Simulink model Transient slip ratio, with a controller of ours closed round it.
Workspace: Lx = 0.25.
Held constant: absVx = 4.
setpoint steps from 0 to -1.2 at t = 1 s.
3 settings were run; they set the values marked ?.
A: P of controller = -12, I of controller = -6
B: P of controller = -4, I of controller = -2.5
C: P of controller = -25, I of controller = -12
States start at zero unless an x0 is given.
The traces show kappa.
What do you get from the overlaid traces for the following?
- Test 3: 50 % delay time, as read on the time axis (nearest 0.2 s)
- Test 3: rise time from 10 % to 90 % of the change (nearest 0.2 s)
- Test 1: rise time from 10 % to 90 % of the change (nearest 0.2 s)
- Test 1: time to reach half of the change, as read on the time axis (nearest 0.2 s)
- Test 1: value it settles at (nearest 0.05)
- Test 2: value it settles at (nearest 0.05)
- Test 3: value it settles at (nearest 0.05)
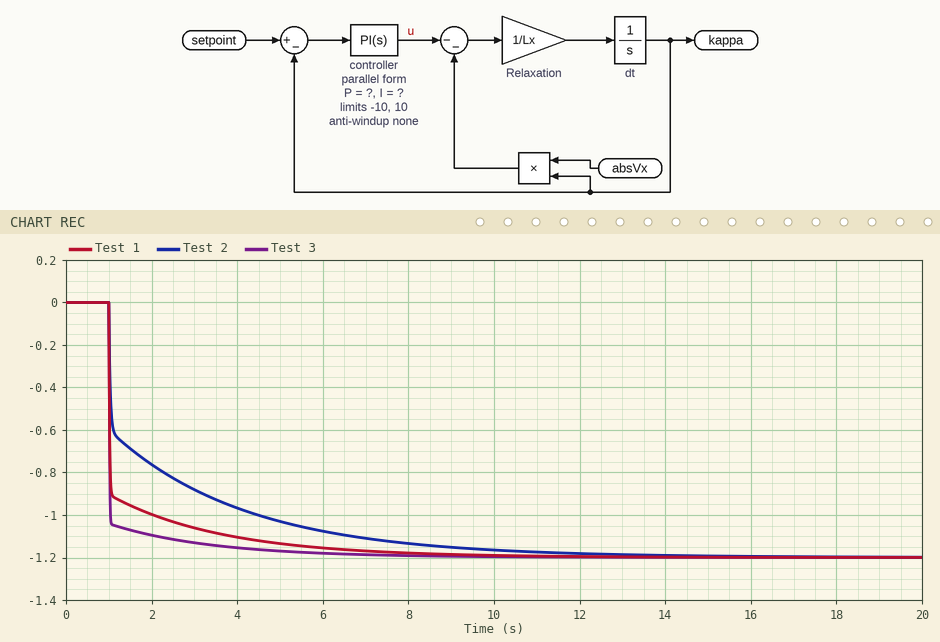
1.0 s
0.6 s
2.4 s
1.0 s
-1.20
-1.20
-1.20
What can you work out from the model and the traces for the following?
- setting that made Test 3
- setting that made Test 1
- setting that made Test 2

C
A
B
